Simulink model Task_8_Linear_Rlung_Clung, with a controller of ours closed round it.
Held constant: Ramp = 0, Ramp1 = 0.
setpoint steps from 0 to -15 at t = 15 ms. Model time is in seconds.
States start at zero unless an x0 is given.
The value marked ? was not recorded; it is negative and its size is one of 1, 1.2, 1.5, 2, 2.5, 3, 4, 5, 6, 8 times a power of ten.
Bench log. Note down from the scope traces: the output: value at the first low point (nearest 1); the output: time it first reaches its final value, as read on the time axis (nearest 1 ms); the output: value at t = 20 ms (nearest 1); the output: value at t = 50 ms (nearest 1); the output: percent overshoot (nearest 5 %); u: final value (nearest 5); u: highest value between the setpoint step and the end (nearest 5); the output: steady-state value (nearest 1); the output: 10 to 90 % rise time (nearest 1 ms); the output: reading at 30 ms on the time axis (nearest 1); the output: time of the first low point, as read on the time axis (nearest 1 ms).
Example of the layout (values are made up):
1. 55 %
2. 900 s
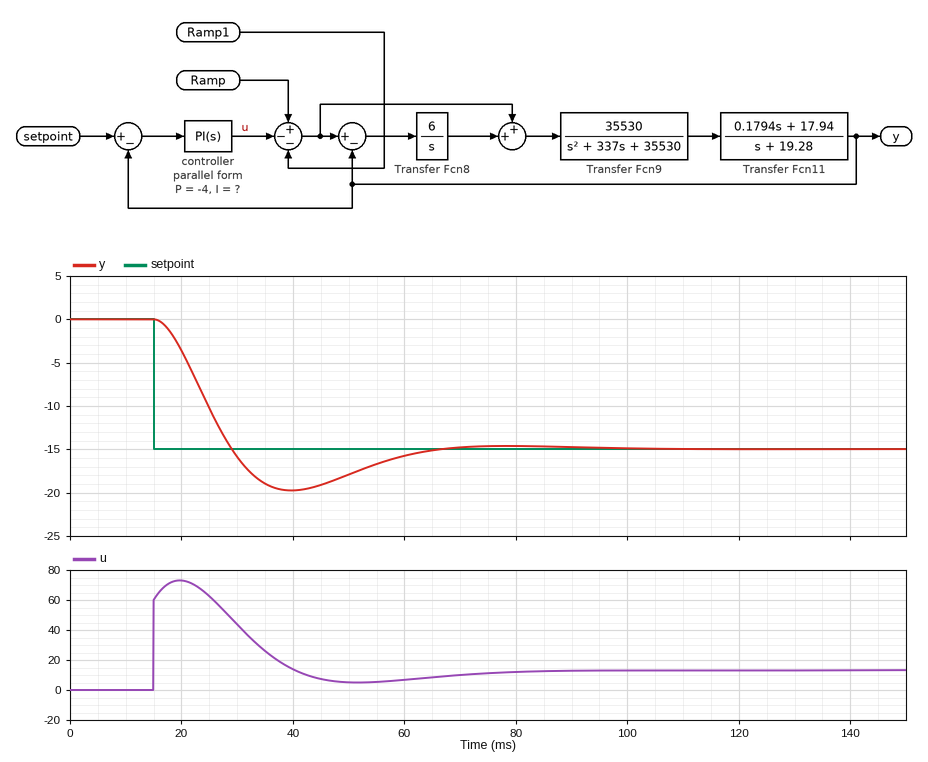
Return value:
1. -20
2. 29 ms
3. -4
4. -18
5. 30 %
6. 15
7. 75
8. -15
9. 10 ms
10. -16
11. 40 ms
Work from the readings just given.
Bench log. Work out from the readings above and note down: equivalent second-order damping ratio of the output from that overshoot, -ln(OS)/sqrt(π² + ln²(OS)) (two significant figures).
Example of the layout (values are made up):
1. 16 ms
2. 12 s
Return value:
1. 0.36
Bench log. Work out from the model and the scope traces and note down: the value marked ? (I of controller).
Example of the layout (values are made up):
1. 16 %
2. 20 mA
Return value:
1. -400
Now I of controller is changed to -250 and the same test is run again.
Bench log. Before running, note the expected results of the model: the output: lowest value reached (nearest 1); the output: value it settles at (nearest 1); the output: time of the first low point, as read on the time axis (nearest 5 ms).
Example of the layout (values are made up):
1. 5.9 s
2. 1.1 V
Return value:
1. -18
2. -15
3. 45 ms
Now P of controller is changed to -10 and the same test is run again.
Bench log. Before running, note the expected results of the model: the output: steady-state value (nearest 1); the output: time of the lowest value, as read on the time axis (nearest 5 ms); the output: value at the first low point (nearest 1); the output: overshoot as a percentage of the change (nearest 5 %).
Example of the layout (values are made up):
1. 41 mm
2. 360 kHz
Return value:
1. -15
2. 30 ms
3. -18
4. 20 %
